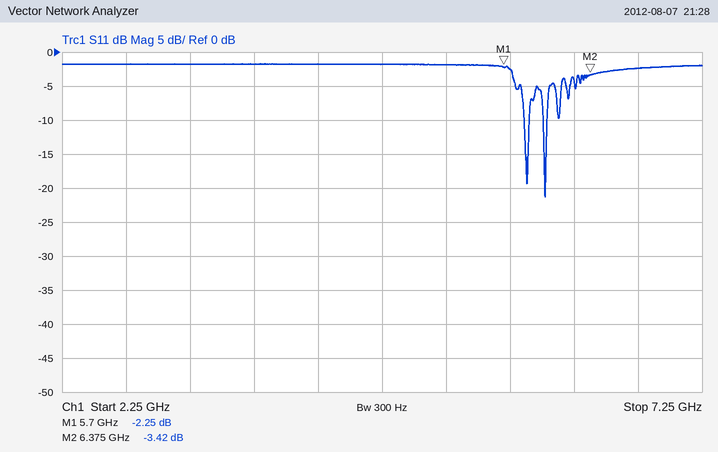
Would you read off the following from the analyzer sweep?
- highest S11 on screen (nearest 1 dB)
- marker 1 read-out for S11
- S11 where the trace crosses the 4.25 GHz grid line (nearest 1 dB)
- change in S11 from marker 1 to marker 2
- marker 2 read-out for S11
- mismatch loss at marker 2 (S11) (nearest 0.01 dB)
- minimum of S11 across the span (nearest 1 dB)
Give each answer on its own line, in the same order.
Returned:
-2 dB
-2.25 dB
-2 dB
-1.17 dB
-3.42 dB
2.64 dB
-21 dB
